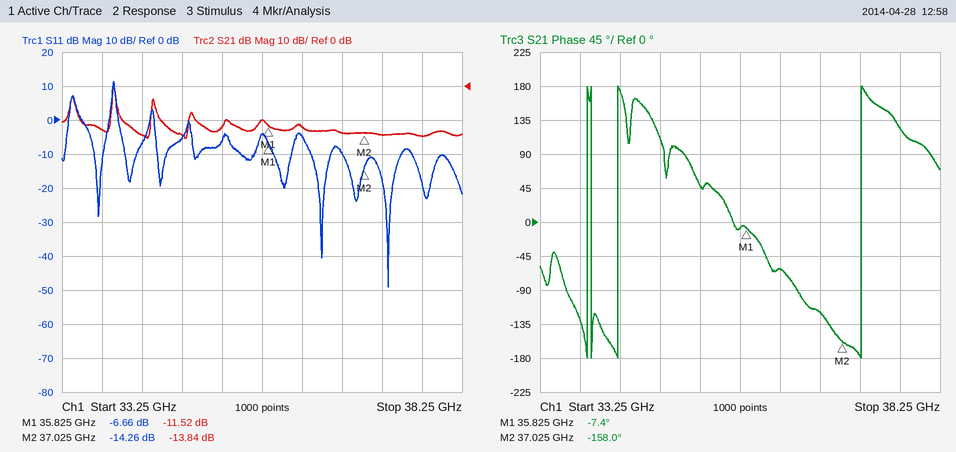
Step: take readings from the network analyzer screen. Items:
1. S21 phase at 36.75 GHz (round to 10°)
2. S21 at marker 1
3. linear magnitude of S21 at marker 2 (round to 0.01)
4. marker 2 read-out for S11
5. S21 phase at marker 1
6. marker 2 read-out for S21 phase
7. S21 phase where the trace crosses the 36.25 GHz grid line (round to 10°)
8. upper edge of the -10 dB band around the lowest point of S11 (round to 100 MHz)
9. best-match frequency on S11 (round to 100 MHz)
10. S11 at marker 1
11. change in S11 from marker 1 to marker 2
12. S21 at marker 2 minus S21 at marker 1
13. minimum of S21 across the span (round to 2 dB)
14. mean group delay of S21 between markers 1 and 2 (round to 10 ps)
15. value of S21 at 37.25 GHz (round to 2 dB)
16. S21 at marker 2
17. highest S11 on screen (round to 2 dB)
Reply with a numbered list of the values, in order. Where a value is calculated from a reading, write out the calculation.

1. -120°
2. -11.52 dB
3. 10^(-13.84/20) ≈ 0.20
4. -14.26 dB
5. -7.4°
6. -158.0°
7. -60°
8. 37.5 GHz
9. 37.3 GHz
10. -6.66 dB
11. -14.26 − (-6.66) = -7.60 dB
12. -13.84 − (-11.52) = -2.32 dB
13. -16 dB
14. −(-158° − (-7.4°))/(360° × 1.2 GHz) ≈ 349 ps, so 350 ps to the nearest 10 ps
15. -14 dB
16. -13.84 dB
17. 12 dB
